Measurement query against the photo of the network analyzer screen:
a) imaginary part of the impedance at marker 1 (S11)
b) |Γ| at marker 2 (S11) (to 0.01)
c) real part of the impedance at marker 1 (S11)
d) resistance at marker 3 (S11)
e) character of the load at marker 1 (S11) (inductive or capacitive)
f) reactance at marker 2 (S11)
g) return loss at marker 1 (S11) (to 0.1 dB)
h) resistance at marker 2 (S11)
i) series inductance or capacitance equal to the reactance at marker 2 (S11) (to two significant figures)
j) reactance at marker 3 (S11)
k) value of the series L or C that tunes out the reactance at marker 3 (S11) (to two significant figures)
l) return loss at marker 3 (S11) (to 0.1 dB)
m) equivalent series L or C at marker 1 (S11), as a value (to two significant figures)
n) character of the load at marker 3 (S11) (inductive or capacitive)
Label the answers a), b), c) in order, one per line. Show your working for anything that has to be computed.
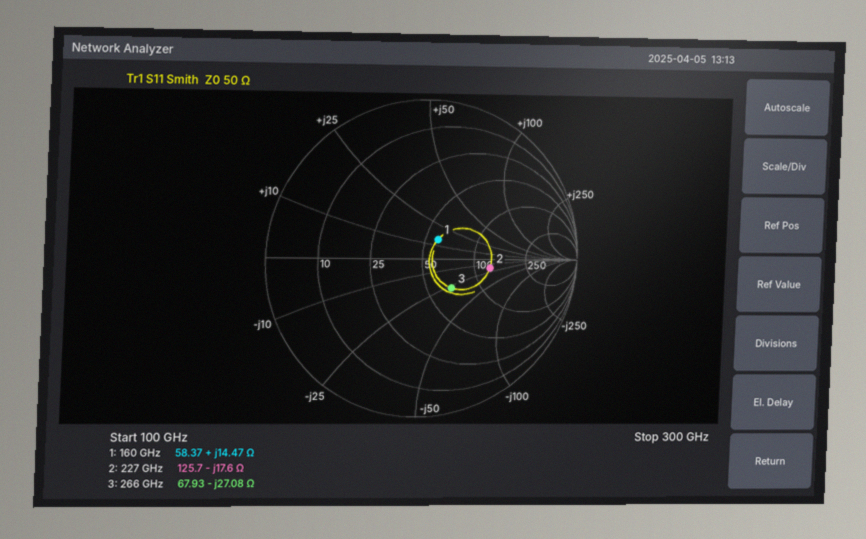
a) +14.47 Ω
b) 0.44
c) 58.37 Ω
d) 67.93 Ω
e) inductive
f) -17.6 Ω
g) 16.3 dB
h) 125.7 Ω
i) C = 1/(2π × 227 GHz × 17.6 Ω) ≈ 40 fF
j) -27.08 Ω
k) L = 27.08 Ω/(2π × 266 GHz) ≈ 16 pH
l) 11.4 dB
m) L = 14.47 Ω/(2π × 160 GHz) ≈ 14 pH
n) capacitive
